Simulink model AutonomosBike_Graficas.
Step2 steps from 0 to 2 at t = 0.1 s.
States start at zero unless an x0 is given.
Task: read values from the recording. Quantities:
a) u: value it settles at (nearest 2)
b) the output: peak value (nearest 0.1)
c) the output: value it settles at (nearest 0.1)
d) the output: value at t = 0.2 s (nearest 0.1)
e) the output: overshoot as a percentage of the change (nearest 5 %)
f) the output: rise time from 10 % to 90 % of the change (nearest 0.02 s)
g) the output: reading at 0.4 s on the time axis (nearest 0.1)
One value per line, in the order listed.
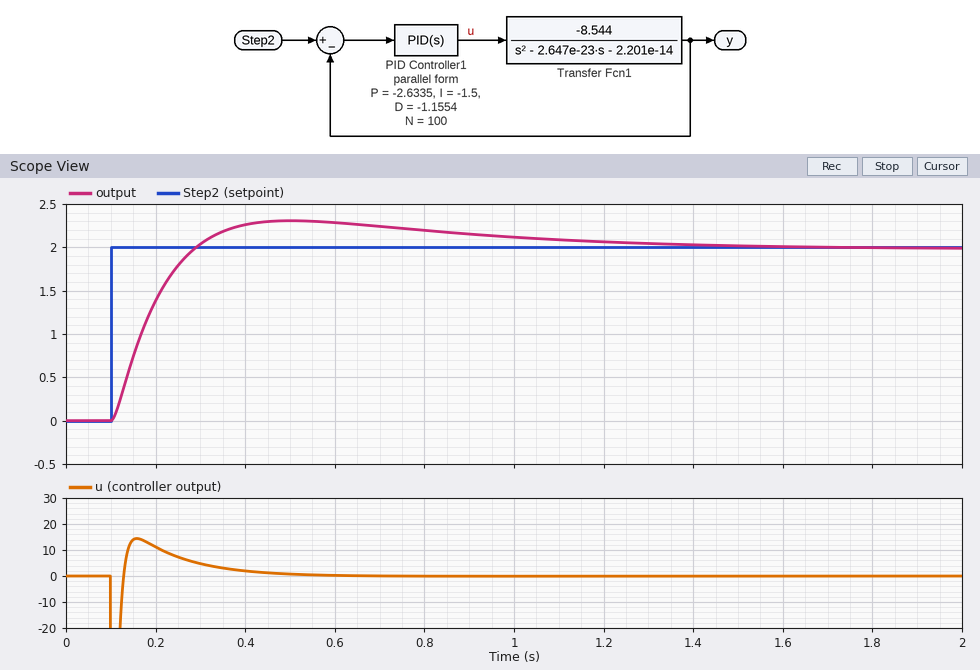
0
2.3
2.0
1.4
15 %
0.14 s
2.3
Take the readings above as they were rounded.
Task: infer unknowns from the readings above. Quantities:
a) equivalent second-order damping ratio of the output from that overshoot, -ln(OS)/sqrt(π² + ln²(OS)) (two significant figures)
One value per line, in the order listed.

0.52
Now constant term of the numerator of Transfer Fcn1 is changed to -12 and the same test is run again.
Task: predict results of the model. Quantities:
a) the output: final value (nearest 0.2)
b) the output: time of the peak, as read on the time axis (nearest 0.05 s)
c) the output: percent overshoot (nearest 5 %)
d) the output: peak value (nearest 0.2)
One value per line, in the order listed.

2.0
0.40 s
10 %
2.2
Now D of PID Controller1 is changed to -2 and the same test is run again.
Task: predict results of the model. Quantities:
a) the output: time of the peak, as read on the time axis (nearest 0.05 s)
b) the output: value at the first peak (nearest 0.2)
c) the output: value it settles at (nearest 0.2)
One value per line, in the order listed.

0.40 s
2.2
2.0
